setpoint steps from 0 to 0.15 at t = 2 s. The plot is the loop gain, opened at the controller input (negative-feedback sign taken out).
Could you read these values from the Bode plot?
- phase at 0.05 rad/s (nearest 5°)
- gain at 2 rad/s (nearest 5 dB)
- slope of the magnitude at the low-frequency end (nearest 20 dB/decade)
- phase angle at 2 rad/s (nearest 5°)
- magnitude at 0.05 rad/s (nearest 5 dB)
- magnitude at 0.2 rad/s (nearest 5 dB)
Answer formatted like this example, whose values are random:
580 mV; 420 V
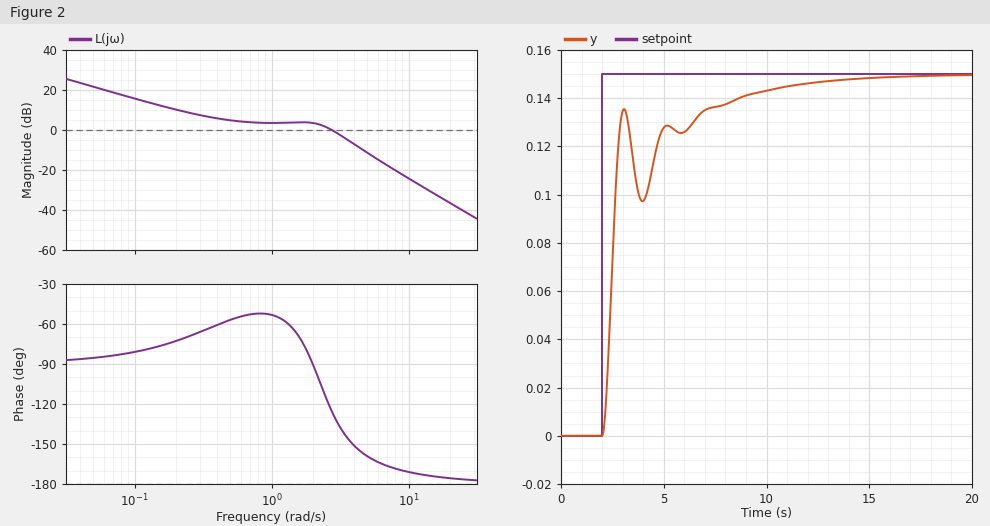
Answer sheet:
-85°; 5 dB; -20 dB/decade; -90°; 20 dB; 10 dB
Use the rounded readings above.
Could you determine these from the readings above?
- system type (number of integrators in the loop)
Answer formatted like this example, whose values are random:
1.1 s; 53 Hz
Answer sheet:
1
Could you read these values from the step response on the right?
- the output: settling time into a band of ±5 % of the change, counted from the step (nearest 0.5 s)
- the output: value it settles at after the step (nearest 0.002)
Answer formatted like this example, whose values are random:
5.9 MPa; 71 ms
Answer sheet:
7.5 s; 0.150
